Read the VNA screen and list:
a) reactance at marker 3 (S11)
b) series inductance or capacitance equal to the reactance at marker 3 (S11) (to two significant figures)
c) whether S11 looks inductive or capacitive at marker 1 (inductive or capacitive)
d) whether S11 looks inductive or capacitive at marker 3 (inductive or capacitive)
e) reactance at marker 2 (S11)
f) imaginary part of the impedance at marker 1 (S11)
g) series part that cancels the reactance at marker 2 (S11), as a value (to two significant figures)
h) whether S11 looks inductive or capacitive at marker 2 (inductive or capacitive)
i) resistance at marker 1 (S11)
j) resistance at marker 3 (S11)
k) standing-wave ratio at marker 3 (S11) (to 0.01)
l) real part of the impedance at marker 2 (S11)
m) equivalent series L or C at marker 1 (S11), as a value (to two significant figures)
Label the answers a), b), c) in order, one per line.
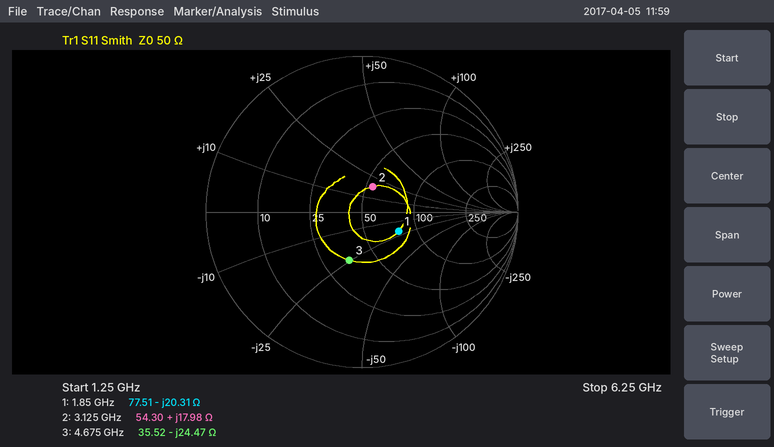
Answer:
a) -24.47 Ω
b) 1.4 pF
c) capacitive
d) capacitive
e) +17.98 Ω
f) -20.31 Ω
g) 2.8 pF
h) inductive
i) 77.51 Ω
j) 35.52 Ω
k) 1.94
l) 54.30 Ω
m) 4.2 pF
